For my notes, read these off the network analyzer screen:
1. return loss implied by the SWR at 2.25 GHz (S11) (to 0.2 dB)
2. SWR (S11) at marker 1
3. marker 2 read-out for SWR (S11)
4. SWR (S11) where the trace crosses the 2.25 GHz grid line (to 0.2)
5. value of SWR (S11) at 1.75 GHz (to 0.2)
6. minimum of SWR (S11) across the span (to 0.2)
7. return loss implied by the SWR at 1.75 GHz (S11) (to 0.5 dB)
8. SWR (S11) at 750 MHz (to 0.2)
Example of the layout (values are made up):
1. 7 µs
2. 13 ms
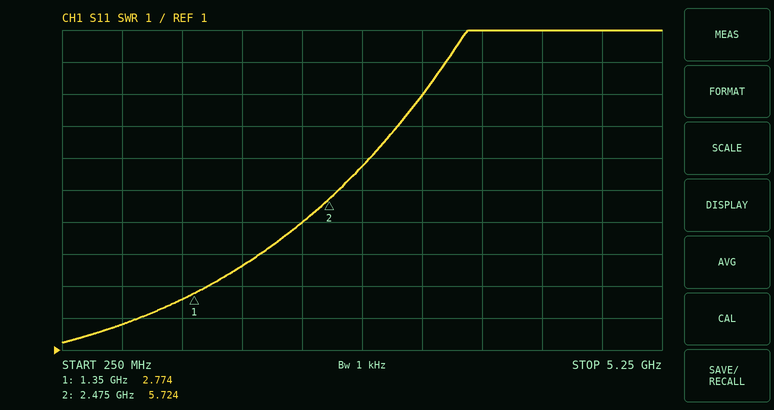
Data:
1. 3.6 dB
2. 2.774
3. 5.724
4. 5.0
5. 3.6
6. 1.2
7. 5.0 dB
8. 1.8
